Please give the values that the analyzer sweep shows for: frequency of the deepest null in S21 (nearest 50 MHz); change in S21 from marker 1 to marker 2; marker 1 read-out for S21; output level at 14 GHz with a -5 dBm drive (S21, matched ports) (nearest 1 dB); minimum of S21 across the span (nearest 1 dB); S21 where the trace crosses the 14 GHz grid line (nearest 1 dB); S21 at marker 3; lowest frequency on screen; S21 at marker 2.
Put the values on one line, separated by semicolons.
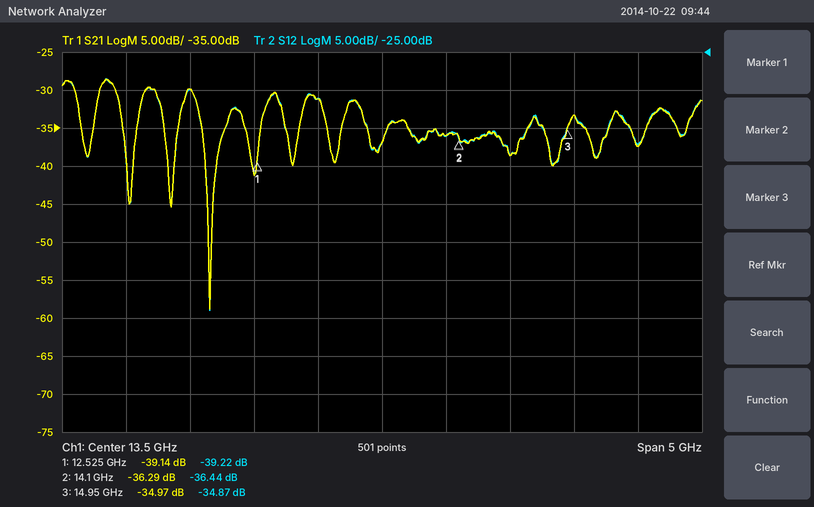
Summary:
12.15 GHz; 2.85 dB; -39.14 dB; -41 dBm; -59 dB; -36 dB; -34.97 dB; 11 GHz; -36.29 dB
